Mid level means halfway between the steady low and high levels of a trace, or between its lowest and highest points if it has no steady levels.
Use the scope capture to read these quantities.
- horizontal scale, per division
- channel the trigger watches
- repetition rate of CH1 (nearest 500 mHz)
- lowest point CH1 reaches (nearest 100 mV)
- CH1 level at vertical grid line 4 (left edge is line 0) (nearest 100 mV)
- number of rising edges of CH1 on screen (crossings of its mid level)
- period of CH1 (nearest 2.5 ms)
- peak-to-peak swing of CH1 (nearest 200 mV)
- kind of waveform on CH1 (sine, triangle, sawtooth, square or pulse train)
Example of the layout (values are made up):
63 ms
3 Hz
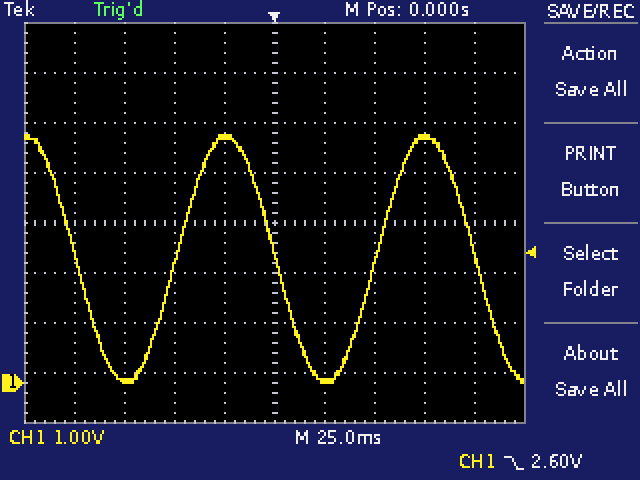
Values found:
25 ms
CH1
10.0 Hz
0.0 V
4.9 V
2
100.0 ms
5.0 V
sine
